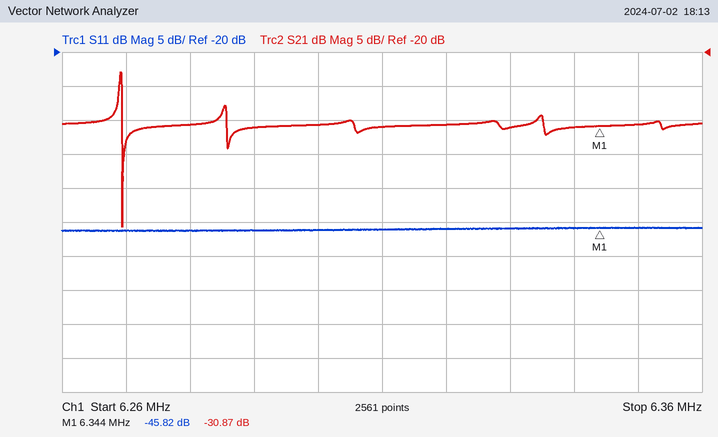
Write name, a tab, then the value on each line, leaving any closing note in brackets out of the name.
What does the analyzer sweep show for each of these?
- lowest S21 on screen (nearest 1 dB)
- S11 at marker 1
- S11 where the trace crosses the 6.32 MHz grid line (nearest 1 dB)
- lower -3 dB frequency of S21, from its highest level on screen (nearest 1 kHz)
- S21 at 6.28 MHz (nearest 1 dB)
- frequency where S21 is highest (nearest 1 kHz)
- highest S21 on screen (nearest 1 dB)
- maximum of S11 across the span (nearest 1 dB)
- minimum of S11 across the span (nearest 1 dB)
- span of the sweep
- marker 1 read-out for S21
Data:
lowest S21 on screen	-46 dB
S11 at marker 1	-45.82 dB
S11 where the trace crosses the 6.32 MHz grid line	-46 dB
lower -3 dB frequency of S21, from its highest level on screen	6.269 MHz
S21 at 6.28 MHz	-31 dB
frequency where S21 is highest	6.269 MHz
highest S21 on screen	-23 dB
maximum of S11 across the span	-46 dB
minimum of S11 across the span	-46 dB
span of the sweep	100 kHz
marker 1 read-out for S21	-30.87 dB
